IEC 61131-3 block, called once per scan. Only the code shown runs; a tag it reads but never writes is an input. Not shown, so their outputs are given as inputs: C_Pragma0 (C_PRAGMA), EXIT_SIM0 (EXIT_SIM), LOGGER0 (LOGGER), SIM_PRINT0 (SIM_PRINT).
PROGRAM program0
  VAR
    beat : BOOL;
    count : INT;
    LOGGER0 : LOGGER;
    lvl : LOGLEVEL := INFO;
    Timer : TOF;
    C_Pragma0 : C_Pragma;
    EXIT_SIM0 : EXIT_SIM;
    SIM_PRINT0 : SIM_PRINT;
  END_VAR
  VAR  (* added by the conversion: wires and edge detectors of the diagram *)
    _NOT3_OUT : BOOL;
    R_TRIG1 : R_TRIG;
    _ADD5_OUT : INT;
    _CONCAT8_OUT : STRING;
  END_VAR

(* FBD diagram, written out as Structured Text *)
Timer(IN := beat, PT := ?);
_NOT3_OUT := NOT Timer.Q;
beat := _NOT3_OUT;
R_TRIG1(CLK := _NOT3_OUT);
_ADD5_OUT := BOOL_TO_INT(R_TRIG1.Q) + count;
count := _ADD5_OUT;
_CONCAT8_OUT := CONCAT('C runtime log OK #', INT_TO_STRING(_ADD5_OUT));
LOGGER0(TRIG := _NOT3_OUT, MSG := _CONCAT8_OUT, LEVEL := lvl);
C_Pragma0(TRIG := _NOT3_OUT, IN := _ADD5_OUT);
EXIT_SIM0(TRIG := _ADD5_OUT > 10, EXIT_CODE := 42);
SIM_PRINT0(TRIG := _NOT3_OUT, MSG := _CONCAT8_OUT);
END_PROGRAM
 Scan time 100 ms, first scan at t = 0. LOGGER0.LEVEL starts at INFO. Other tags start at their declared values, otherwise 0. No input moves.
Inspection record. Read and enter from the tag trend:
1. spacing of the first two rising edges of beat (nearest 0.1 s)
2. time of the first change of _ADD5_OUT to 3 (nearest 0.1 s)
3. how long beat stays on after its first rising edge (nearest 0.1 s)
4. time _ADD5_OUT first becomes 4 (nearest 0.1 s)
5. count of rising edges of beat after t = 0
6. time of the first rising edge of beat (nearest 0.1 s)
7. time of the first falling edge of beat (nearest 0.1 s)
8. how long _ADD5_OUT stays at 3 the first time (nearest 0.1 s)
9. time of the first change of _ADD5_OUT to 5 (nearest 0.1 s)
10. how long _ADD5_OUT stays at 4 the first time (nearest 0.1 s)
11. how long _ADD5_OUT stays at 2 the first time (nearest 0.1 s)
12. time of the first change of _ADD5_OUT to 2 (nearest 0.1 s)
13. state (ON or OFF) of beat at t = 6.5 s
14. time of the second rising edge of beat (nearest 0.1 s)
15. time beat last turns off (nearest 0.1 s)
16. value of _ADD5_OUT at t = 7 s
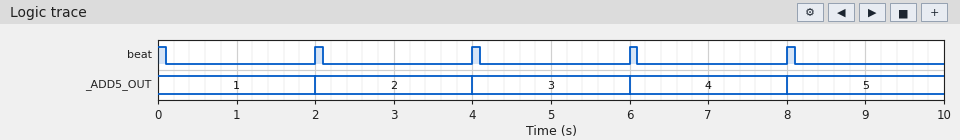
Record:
2.0 s
4.0 s
0.1 s
6.0 s
4
2.0 s
0.1 s
2.0 s
8.0 s
2.0 s
2.0 s
2.0 s
OFF
4.0 s
8.1 s
4
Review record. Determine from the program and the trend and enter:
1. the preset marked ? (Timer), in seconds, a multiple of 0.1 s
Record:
1.8 s
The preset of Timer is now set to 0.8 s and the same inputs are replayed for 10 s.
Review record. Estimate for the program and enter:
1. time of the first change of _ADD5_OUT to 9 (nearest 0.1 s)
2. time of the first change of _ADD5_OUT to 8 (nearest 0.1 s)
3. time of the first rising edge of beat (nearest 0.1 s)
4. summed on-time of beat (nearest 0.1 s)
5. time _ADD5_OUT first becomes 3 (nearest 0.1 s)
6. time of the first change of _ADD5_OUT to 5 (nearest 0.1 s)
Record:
8.0 s
7.0 s
1.0 s
1.0 s
2.0 s
4.0 s
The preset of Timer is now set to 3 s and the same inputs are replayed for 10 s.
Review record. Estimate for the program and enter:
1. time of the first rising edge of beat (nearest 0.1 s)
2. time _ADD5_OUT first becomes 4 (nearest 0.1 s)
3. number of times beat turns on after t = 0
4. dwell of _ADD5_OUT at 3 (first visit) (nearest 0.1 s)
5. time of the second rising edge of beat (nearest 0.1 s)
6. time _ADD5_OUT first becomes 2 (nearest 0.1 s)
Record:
3.2 s
9.6 s
3
3.2 s
6.4 s
3.2 s
